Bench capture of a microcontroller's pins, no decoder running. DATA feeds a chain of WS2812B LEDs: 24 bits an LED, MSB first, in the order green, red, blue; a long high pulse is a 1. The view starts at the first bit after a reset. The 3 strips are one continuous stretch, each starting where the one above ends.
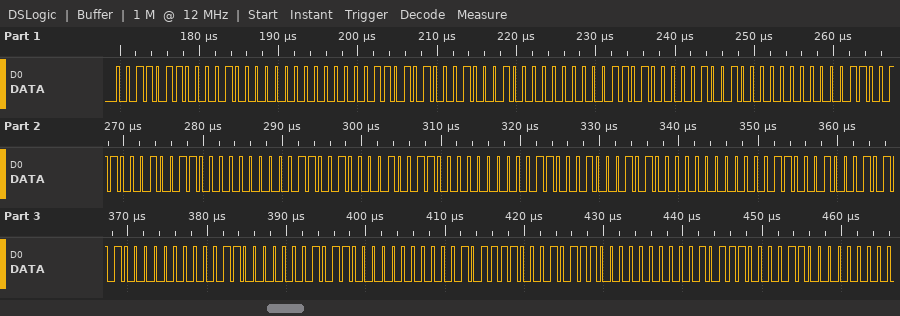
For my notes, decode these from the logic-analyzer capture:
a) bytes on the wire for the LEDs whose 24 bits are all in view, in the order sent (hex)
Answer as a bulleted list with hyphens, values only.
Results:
- 36 10 00 35 11 00 34 12 00 33 13 00 32 13 00 31 14 00 31 15 00 30 16 00 2F 17 00
